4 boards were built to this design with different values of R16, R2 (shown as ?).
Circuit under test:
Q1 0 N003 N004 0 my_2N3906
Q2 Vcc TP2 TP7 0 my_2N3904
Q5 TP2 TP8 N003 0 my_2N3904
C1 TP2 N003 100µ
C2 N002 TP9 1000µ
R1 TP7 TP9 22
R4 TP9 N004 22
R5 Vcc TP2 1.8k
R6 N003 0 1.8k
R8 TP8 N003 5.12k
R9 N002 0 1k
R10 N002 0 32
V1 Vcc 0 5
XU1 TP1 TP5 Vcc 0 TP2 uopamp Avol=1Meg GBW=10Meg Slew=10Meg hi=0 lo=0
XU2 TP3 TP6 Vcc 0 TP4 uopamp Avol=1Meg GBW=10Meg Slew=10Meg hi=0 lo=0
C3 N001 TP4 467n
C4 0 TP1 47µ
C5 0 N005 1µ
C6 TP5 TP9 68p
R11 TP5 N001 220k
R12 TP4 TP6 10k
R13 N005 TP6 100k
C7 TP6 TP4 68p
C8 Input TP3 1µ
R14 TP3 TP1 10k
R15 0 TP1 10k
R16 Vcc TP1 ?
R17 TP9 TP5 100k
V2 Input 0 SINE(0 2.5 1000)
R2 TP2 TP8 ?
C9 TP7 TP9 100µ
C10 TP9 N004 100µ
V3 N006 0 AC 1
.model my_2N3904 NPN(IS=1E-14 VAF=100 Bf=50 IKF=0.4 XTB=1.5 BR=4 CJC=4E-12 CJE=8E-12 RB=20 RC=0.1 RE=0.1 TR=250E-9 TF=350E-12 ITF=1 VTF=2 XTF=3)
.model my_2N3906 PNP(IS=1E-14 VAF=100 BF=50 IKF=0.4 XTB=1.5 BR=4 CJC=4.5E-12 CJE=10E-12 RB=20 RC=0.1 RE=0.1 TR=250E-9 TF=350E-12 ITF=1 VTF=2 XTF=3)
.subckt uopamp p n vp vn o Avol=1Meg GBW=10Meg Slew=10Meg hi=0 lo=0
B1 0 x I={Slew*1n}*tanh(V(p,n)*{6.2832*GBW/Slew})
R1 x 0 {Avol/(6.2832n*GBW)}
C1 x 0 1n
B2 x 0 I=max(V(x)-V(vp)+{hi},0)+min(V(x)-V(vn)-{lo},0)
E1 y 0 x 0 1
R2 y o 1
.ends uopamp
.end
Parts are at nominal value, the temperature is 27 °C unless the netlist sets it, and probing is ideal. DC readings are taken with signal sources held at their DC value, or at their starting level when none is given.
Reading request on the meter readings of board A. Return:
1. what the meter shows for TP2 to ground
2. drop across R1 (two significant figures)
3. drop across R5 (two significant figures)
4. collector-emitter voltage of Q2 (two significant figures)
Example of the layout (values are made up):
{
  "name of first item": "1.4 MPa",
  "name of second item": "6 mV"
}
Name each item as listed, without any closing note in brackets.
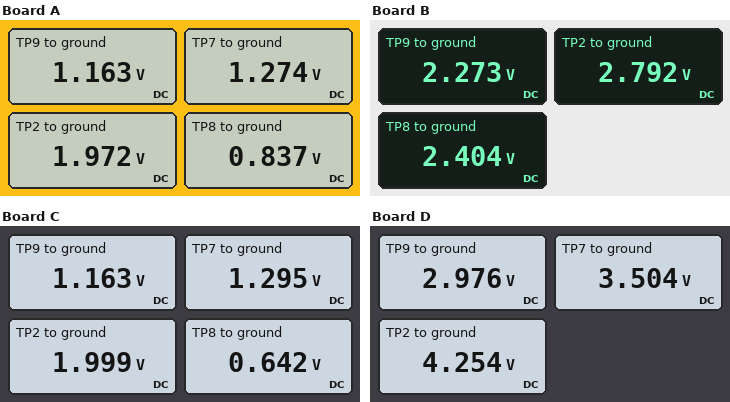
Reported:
{
  "what the meter shows for TP2 to ground": "1.972 V",
  "drop across R1": "110 mV",
  "drop across R5": "3.0 V",
  "collector-emitter voltage of Q2": "3.7 V"
}
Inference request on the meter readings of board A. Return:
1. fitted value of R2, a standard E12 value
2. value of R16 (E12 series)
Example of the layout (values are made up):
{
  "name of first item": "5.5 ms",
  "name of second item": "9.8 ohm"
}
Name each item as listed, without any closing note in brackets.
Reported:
{
  "fitted value of R2, a standard E12 value": "12 kΩ",
  "value of R16": "33 kΩ"
}
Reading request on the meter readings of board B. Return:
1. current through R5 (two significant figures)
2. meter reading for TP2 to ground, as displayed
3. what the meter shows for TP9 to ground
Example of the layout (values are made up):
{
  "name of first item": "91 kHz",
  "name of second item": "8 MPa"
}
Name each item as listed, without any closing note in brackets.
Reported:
{
  "current through R5": "1.2 mA",
  "meter reading for TP2 to ground, as displayed": "2.792 V",
  "what the meter shows for TP9 to ground": "2.273 V"
}
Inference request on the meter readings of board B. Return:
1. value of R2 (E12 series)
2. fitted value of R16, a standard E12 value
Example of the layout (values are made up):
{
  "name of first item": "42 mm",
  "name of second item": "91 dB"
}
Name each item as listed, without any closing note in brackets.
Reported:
{
  "value of R2": "2.7 kΩ",
  "fitted value of R16, a standard E12 value": "12 kΩ"
}
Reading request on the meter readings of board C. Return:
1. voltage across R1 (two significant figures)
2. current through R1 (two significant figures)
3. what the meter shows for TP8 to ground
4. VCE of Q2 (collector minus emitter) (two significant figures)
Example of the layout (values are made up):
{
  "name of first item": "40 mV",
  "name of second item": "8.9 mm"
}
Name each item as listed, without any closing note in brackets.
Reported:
{
  "voltage across R1": "130 mV",
  "current through R1": "6.0 mA",
  "what the meter shows for TP8 to ground": "0.642 V",
  "VCE of Q2 (collector minus emitter)": "3.7 V"
}
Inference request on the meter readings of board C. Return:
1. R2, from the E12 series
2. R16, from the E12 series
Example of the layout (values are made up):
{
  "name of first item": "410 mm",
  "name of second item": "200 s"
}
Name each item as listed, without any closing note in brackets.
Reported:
{
  "R2, from the E12 series": "22 kΩ",
  "R16, from the E12 series": "33 kΩ"
}
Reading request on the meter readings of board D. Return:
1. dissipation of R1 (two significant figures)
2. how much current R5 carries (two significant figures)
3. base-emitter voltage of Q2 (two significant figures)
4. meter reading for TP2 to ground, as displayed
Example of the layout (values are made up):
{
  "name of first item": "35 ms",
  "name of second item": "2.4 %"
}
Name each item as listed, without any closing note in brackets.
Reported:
{
  "dissipation of R1": "13 mW",
  "how much current R5 carries": "410 µA",
  "base-emitter voltage of Q2": "750 mV",
  "meter reading for TP2 to ground, as displayed": "4.254 V"
}
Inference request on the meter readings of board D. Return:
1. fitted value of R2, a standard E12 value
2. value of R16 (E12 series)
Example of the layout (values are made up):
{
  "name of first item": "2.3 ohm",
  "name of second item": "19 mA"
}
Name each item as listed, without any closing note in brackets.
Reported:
{
  "fitted value of R2, a standard E12 value": "15 kΩ",
  "value of R16": "6.8 kΩ"
}
